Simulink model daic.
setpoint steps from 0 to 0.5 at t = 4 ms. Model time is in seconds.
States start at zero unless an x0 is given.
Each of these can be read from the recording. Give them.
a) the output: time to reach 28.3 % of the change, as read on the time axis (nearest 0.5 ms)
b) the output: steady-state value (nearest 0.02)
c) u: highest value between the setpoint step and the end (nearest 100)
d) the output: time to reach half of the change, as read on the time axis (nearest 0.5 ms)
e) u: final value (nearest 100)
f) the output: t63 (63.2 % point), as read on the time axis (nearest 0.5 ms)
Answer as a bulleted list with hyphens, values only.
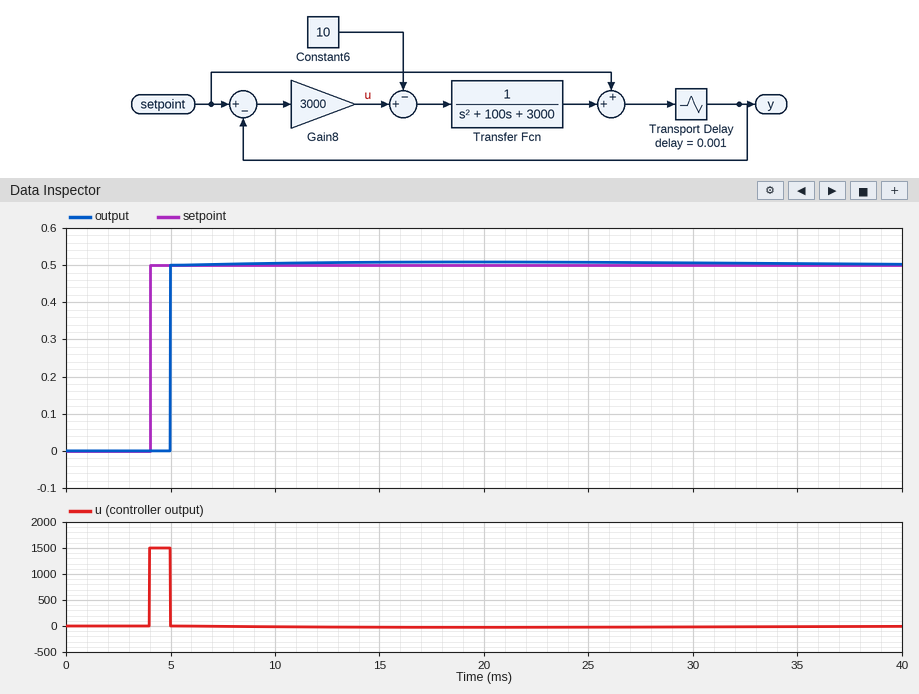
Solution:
- 5.0 ms
- 0.50
- 1500
- 5.0 ms
- 0
- 5.0 ms
